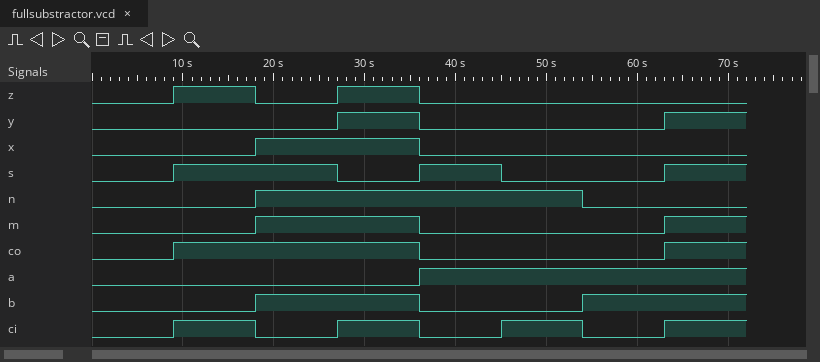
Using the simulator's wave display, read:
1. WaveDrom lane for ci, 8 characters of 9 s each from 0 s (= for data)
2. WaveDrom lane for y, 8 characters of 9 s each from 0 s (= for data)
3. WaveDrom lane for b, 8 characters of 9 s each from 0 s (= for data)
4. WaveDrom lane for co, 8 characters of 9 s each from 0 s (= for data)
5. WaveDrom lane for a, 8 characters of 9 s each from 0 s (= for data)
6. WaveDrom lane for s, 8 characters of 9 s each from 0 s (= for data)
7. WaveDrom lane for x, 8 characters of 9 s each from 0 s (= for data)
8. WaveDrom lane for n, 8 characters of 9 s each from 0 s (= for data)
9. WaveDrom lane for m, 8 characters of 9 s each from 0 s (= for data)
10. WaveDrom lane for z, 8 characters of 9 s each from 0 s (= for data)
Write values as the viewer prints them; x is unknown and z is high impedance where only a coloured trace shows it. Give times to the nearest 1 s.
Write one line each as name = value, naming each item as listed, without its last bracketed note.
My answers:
WaveDrom lane for ci, 8 characters of 9 s each from 0 s = {name: 'ci', wave: '01010101'}
WaveDrom lane for y, 8 characters of 9 s each from 0 s = {name: 'y', wave: '0..10..1'}
WaveDrom lane for b, 8 characters of 9 s each from 0 s = {name: 'b', wave: '0.1.0.1.'}
WaveDrom lane for co, 8 characters of 9 s each from 0 s = {name: 'co', wave: '01..0..1'}
WaveDrom lane for a, 8 characters of 9 s each from 0 s = {name: 'a', wave: '0...1...'}
WaveDrom lane for s, 8 characters of 9 s each from 0 s = {name: 's', wave: '01.010.1'}
WaveDrom lane for x, 8 characters of 9 s each from 0 s = {name: 'x', wave: '0.1.0...'}
WaveDrom lane for n, 8 characters of 9 s each from 0 s = {name: 'n', wave: '0.1...0.'}
WaveDrom lane for m, 8 characters of 9 s each from 0 s = {name: 'm', wave: '0.1.0..1'}
WaveDrom lane for z, 8 characters of 9 s each from 0 s = {name: 'z', wave: '01010...'}
